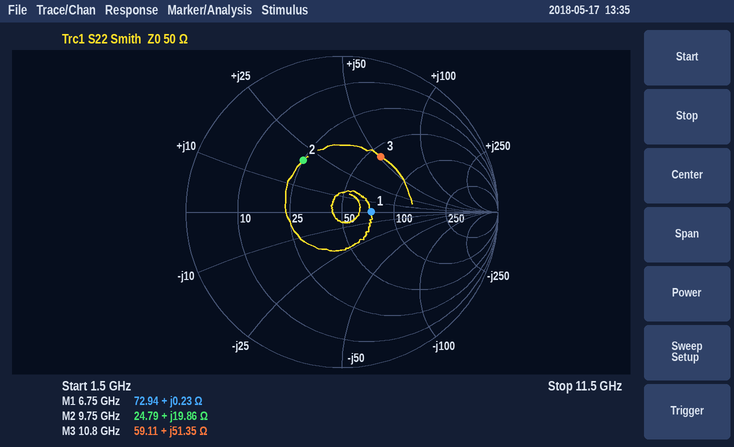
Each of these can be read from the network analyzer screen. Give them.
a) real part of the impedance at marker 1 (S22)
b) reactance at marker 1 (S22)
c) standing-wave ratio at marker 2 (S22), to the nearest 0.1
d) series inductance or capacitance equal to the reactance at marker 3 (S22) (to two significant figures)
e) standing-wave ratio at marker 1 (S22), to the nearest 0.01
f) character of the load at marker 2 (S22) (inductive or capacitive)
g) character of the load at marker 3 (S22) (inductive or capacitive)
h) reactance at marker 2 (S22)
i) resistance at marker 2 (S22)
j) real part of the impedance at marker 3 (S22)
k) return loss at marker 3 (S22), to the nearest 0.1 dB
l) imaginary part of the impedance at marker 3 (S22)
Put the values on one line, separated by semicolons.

72.94 Ω; +0.23 Ω; 2.4; 760 pH; 1.46; inductive; inductive; +19.86 Ω; 24.79 Ω; 59.11 Ω; 7.3 dB; +51.35 Ω
